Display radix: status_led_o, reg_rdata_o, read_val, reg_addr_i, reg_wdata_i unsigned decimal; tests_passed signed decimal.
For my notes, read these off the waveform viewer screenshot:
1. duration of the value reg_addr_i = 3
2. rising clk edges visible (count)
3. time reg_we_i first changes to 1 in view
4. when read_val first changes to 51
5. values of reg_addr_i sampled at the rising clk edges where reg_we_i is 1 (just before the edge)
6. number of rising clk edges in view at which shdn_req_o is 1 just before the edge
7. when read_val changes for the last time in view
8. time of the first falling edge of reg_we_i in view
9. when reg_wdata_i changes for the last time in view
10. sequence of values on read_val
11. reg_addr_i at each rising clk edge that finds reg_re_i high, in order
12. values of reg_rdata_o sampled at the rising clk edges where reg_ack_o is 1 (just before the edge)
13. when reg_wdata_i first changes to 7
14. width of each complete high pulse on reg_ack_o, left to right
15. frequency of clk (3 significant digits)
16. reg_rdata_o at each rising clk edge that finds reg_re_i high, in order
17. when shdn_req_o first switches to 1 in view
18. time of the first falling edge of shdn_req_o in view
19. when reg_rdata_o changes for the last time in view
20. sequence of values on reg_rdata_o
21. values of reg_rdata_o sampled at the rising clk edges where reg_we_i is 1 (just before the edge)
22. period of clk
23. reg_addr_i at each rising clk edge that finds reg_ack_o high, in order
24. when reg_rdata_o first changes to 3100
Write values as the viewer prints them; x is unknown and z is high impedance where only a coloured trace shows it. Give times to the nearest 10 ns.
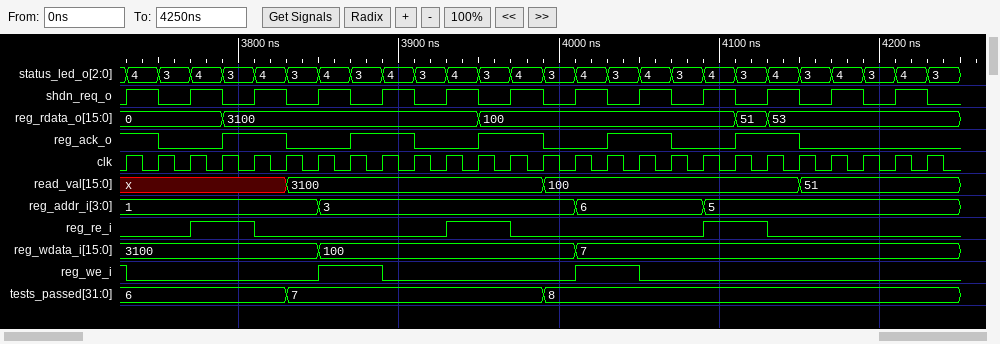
160 ns
26
3850 ns
4150 ns
1, 3, 3, 6, 6
13
4150 ns
3730 ns
4010 ns
x, 3100, 100, 51
1, 1, 3, 3, 5, 5
0, 0, 3100, 3100, 3100, 3100, 100, 100, 100, 100, 51, 53
4010 ns
40 ns, 40 ns, 40 ns, 40 ns, 40 ns
50.0 MHz
0, 3100, 3100, 100, 100, 51
3730 ns
3750 ns
4130 ns
0, 3100, 100, 51, 53
0, 3100, 3100, 100, 100
20 ns
1, 1, 1, 1, 3, 3, 3, 3, 6, 6, 5, 5
3790 ns
